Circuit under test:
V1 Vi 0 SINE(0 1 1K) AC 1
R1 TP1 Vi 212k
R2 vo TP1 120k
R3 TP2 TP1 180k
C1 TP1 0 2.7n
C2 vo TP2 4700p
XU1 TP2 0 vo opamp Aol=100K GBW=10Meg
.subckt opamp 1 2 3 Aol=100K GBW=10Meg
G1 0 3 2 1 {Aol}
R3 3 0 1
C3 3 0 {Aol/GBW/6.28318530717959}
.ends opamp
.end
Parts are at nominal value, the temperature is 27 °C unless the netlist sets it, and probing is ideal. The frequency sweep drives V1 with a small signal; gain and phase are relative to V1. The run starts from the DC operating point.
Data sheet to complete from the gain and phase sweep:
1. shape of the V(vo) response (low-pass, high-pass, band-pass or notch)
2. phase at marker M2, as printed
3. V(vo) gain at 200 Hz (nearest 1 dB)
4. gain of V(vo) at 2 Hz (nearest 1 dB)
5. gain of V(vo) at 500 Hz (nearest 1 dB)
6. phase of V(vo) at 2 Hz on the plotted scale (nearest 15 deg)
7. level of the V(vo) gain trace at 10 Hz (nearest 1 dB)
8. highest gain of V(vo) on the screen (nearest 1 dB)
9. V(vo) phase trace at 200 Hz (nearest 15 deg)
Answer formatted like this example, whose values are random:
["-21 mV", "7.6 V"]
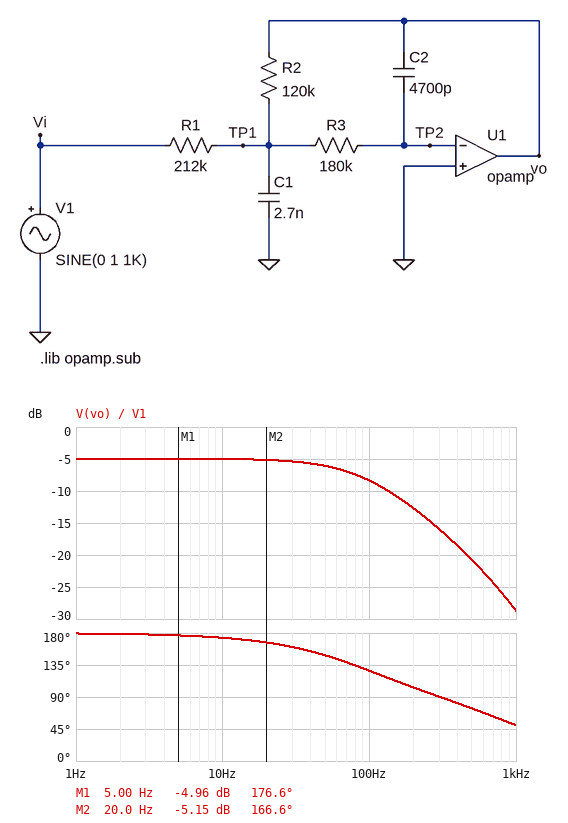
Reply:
["low-pass", "166.6 deg", "-13 dB", "-5 dB", "-21 dB", "180 deg", "-5 dB", "-5 dB", "105 deg"]
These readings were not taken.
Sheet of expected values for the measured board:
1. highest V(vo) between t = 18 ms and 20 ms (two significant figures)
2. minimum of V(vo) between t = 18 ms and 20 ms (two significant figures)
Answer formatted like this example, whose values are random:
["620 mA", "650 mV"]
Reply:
["37 mV", "-37 mV"]
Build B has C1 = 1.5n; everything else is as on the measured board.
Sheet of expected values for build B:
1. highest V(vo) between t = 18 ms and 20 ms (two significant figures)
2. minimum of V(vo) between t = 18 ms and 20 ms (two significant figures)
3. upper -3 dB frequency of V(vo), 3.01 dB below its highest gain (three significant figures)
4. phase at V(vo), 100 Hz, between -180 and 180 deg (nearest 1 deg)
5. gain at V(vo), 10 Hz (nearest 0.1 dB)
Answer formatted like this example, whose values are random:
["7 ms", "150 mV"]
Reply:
["44 mV", "-44 mV", "88.0 Hz", "128 deg", "-5.0 dB"]
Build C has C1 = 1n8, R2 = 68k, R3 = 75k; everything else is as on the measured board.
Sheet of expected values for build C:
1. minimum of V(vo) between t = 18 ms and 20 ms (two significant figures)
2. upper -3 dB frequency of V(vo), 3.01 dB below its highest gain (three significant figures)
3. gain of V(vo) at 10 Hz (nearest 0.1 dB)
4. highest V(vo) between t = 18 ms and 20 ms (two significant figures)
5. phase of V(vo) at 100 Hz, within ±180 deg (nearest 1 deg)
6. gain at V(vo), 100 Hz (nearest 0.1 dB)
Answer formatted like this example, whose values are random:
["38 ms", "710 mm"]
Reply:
["-64 mV", "218 Hz", "-9.9 dB", "64 mV", "153 deg", "-10.7 dB"]
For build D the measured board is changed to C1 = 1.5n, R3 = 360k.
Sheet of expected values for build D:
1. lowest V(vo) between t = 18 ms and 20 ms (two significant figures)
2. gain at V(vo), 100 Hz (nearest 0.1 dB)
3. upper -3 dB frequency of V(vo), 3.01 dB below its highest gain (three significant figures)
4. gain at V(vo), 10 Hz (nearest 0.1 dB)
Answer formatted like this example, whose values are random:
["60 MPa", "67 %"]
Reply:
["-25 mV", "-11.8 dB", "51.0 Hz", "-5.1 dB"]
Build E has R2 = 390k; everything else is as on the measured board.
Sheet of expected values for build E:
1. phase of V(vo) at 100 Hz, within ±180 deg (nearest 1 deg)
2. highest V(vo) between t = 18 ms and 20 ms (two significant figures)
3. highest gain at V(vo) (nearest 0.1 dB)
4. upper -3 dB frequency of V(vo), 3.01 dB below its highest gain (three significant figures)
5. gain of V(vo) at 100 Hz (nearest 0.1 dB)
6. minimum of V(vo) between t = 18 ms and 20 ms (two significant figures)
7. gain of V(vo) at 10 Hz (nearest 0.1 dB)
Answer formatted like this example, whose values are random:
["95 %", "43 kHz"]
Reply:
["104 deg", "42 mV", "5.3 dB", "39.5 Hz", "-3.5 dB", "-43 mV", "5.0 dB"]
